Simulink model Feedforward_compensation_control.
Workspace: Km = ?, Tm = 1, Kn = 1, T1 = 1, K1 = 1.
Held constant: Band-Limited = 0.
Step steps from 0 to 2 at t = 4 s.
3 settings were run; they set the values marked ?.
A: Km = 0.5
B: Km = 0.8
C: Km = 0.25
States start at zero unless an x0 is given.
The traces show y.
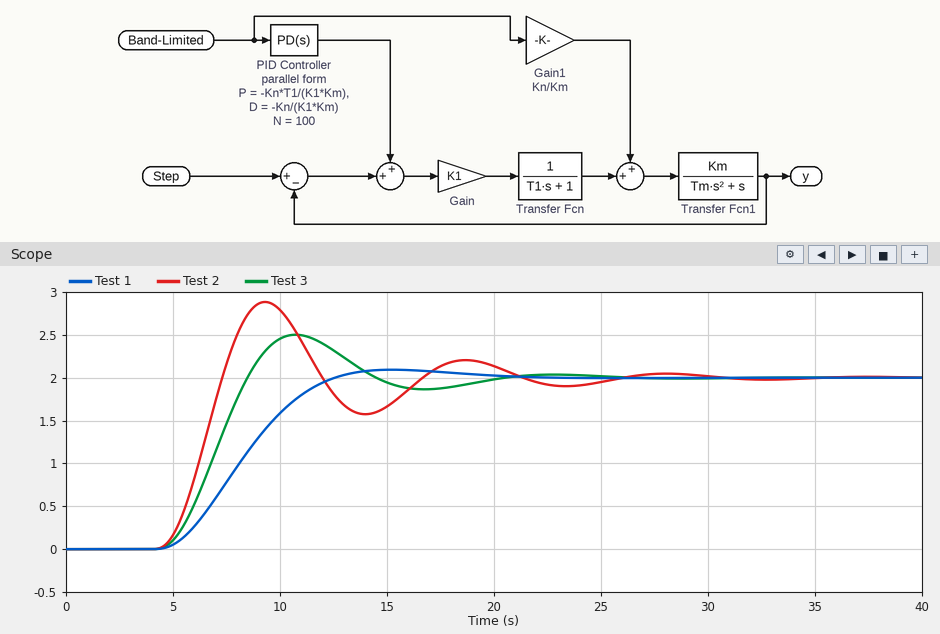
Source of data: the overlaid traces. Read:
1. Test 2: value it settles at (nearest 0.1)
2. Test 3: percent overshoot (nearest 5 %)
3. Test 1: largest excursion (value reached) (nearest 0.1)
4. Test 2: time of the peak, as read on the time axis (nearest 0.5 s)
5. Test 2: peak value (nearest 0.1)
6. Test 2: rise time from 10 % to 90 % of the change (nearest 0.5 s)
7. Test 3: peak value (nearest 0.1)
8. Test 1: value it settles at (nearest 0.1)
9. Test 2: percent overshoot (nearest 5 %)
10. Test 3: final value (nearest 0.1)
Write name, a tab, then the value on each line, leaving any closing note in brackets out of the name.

Test 2: value it settles at	2.0
Test 3: percent overshoot	25 %
Test 1: largest excursion (value reached)	2.1
Test 2: time of the peak, as read on the time axis	9.5 s
Test 2: peak value	2.9
Test 2: rise time from 10 % to 90 % of the change	2.0 s
Test 3: peak value	2.5
Test 1: value it settles at	2.0
Test 2: percent overshoot	45 %
Test 3: final value	2.0
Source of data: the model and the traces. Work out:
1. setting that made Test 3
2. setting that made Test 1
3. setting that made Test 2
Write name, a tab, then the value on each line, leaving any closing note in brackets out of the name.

setting that made Test 3	A
setting that made Test 1	C
setting that made Test 2	B
